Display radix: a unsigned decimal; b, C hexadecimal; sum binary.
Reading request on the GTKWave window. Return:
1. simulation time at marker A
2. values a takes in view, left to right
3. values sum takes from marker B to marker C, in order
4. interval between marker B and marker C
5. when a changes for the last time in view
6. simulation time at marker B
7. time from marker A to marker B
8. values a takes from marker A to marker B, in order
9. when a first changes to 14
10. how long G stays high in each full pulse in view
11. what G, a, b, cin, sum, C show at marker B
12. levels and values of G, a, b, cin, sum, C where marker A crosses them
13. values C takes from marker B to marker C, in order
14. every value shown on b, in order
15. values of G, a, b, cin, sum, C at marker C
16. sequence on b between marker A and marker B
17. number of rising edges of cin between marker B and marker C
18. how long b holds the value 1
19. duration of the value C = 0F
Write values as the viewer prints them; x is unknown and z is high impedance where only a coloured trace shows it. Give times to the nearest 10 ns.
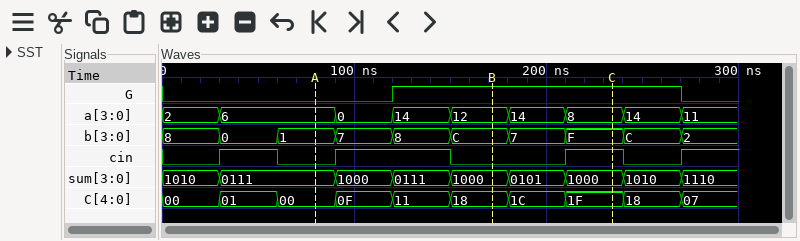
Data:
80 ns
2, 6, 0, 14, 12, 14, 8, 14, 11
1000, 0101, 1000
60 ns
270 ns
170 ns
90 ns
6, 0, 14, 12
120 ns
150 ns
G=1, a=12, b=C, cin=0, sum=1000, C=18
G=0, a=6, b=1, cin=0, sum=0111, C=00
18, 1C, 1F
8, 0, 1, 7, 8, C, 7, F, C, 2
G=1, a=8, b=F, cin=1, sum=1000, C=1F
1, 7, 8, C
1
30 ns
30 ns
